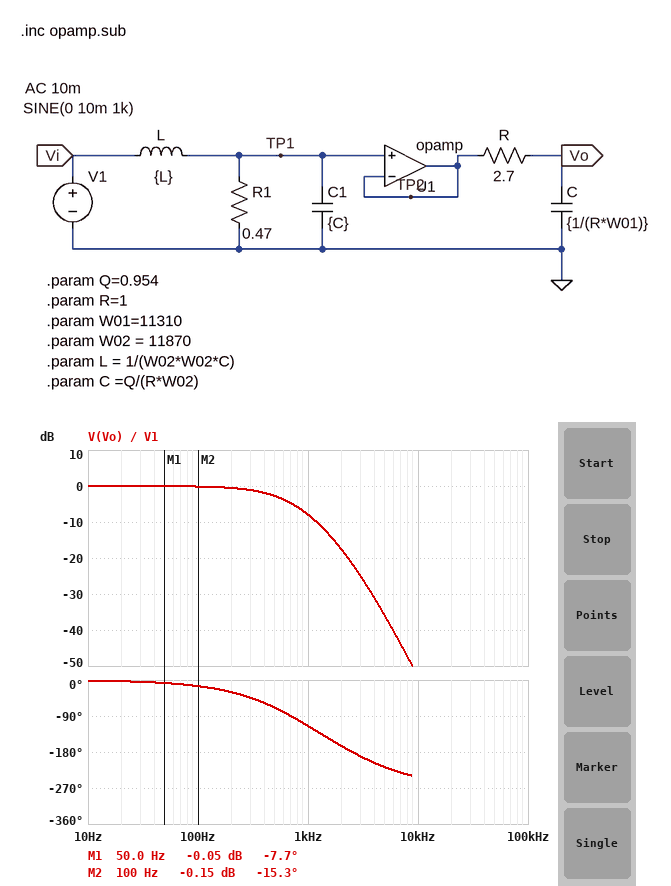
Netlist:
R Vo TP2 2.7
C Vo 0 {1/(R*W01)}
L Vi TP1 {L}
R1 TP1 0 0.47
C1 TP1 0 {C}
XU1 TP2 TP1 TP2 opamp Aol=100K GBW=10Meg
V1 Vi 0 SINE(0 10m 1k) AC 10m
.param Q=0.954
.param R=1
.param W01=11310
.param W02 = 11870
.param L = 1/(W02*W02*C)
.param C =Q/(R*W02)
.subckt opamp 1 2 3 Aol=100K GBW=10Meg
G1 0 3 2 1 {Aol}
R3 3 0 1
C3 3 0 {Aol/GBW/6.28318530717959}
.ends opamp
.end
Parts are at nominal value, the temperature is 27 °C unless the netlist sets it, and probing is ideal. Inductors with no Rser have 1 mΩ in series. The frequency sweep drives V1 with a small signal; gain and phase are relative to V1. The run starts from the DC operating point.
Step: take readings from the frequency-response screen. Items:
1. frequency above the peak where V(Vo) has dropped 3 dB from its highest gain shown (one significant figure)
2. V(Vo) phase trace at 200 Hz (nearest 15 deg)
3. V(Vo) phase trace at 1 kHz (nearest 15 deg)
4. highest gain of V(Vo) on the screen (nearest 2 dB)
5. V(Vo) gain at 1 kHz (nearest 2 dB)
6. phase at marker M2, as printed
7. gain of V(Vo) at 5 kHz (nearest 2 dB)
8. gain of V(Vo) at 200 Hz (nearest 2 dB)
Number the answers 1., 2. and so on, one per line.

1. 500 Hz
2. -30 deg
3. -120 deg
4. 0 dB
5. -8 dB
6. -15.3 deg
7. -36 dB
8. 0 dB
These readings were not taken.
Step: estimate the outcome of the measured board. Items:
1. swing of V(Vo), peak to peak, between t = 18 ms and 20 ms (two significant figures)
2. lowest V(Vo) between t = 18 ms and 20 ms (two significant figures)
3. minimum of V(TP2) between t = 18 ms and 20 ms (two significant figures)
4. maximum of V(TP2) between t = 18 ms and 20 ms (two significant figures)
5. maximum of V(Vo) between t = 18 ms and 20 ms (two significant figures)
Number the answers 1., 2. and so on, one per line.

1. 8.0 mV
2. -4.0 mV
3. -7.2 mV
4. 7.2 mV
5. 4.0 mV
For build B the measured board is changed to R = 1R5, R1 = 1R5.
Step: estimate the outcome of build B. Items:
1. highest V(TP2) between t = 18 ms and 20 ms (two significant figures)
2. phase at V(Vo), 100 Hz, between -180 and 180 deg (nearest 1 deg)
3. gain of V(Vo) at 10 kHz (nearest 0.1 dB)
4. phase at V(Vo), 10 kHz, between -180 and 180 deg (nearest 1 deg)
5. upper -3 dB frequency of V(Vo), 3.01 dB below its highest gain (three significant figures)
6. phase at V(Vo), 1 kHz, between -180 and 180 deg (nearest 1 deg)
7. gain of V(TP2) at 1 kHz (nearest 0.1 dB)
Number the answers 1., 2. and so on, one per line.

1. 12 mV
2. -7 deg
3. -47.2 dB
4. 105 deg
5. 1.97 kHz
6. -67 deg
7. 1.8 dB
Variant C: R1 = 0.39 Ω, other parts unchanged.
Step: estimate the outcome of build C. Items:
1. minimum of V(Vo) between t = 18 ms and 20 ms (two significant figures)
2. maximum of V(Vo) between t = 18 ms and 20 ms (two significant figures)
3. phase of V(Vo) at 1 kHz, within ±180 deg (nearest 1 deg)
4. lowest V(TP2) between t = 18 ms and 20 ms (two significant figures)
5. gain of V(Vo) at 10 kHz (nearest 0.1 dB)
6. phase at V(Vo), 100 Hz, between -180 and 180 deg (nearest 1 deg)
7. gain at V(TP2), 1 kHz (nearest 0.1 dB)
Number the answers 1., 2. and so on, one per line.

1. -3.5 mV
2. 3.5 mV
3. -119 deg
4. -6.3 mV
5. -53.2 dB
6. -17 deg
7. -4.1 dB
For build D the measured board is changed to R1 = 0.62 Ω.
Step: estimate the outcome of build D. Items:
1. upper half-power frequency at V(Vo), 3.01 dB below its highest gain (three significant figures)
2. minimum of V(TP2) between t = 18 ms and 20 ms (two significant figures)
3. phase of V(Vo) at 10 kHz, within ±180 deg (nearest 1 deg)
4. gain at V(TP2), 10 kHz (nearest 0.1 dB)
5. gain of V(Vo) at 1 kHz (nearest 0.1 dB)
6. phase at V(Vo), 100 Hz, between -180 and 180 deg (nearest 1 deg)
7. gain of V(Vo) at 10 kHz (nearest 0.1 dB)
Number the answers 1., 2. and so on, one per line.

1. 604 Hz
2. -8.7 mV
3. 112 deg
4. -29.1 dB
5. -6.3 dB
6. -14 deg
7. -52.6 dB
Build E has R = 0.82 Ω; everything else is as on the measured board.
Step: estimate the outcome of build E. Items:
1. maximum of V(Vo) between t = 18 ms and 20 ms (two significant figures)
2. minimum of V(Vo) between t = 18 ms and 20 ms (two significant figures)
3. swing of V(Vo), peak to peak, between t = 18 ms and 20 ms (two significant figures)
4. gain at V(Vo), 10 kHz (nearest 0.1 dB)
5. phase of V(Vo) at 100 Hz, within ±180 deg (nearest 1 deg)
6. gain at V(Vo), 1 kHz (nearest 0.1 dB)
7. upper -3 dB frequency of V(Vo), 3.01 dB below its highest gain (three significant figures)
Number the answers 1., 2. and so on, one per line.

1. 6.6 mV
2. -6.6 mV
3. 13 mV
4. -42.8 dB
5. -9 deg
6. -3.6 dB
7. 895 Hz
